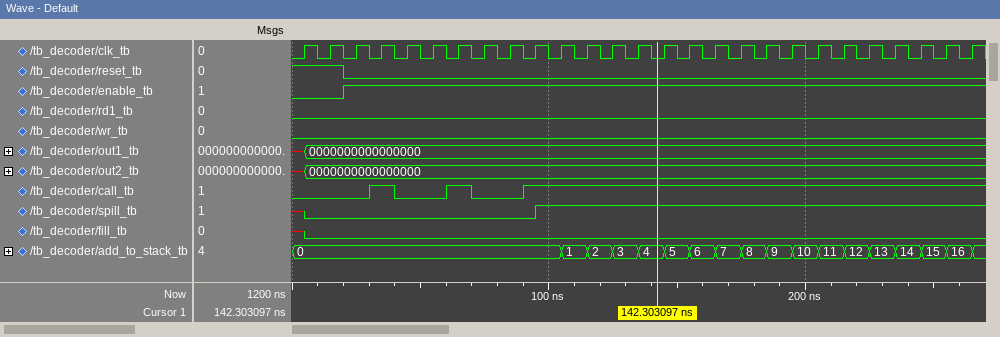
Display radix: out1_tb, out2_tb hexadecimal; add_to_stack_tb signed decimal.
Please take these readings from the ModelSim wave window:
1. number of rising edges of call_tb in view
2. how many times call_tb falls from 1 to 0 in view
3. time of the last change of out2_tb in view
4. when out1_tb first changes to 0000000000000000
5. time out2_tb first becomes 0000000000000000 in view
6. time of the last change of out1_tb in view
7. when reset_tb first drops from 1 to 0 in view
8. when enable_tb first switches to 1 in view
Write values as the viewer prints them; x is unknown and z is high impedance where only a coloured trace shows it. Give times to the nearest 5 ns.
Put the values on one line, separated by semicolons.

3; 2; 5 ns; 5 ns; 5 ns; 5 ns; 20 ns; 20 ns
